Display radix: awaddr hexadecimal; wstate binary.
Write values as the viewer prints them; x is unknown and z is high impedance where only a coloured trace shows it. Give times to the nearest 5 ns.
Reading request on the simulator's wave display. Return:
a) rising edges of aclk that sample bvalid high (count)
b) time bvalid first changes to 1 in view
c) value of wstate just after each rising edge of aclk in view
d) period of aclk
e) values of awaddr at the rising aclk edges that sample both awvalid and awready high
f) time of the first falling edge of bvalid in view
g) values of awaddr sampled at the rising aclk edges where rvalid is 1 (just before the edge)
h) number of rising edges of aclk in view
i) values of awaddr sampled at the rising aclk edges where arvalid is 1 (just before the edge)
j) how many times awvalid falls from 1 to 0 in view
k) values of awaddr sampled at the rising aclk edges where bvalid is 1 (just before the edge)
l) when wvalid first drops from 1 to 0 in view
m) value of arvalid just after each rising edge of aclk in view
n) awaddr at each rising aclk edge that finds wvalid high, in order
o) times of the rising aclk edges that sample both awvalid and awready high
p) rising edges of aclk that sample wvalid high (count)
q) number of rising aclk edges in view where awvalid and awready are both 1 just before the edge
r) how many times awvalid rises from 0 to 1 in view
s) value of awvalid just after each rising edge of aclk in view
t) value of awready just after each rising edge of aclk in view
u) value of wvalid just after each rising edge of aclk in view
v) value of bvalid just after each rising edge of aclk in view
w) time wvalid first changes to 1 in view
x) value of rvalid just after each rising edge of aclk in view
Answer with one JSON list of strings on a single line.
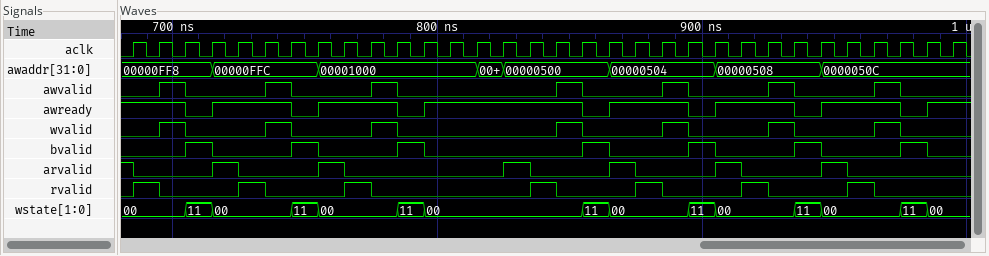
["7", "705 ns", "00, 00, 11, 00, 00, 00, 11, 00, 00, 00, 11, 00, 00, 00, 00, 00, 00, 11, 00, 00, 00, 11, 00, 00, 00, 11, 00, 00, 00, 11, 00, 00", "10 ns", "00000FF8, 00000FFC, 00001000, 00000500, 00000504, 00000508, 0000050C", "715 ns", "00000FF8, 00000FFC, 00001000, 00000500, 00000504, 00000508, 0000050C", "32", "00000FF8, 00000FFC, 00001000, 00000500, 00000504, 00000508, 0000050C", "7", "00000FF8, 00000FFC, 00001000, 00000500, 00000504, 00000508, 0000050C", "705 ns", "0 0 0 1 0 0 0 1 0 0 0 0 0 0 1 0 0 0 1 0 0 0 1 0 0 0 1 0 0 0 0 0", "00000FF8, 00000FFC, 00001000, 00000500, 00000504, 00000508, 0000050C", "705 ns, 745 ns, 785 ns, 855 ns, 895 ns, 935 ns, 975 ns", "7", "7", "7", "0 1 0 0 0 1 0 0 0 1 0 0 0 0 0 0 1 0 0 0 1 0 0 0 1 0 0 0 1 0 0 0", "1 1 0 1 1 1 0 1 1 1 0 1 1 1 1 1 1 0 1 1 1 0 1 1 1 0 1 1 1 0 1 1", "0 1 0 0 0 1 0 0 0 1 0 0 0 0 0 0 1 0 0 0 1 0 0 0 1 0 0 0 1 0 0 0", "0 0 1 0 0 0 1 0 0 0 1 0 0 0 0 0 0 1 0 0 0 1 0 0 0 1 0 0 0 1 0 0", "695 ns", "1 0 0 0 1 0 0 0 1 0 0 0 0 0 0 1 0 0 0 1 0 0 0 1 0 0 0 1 0 0 0 0"]
